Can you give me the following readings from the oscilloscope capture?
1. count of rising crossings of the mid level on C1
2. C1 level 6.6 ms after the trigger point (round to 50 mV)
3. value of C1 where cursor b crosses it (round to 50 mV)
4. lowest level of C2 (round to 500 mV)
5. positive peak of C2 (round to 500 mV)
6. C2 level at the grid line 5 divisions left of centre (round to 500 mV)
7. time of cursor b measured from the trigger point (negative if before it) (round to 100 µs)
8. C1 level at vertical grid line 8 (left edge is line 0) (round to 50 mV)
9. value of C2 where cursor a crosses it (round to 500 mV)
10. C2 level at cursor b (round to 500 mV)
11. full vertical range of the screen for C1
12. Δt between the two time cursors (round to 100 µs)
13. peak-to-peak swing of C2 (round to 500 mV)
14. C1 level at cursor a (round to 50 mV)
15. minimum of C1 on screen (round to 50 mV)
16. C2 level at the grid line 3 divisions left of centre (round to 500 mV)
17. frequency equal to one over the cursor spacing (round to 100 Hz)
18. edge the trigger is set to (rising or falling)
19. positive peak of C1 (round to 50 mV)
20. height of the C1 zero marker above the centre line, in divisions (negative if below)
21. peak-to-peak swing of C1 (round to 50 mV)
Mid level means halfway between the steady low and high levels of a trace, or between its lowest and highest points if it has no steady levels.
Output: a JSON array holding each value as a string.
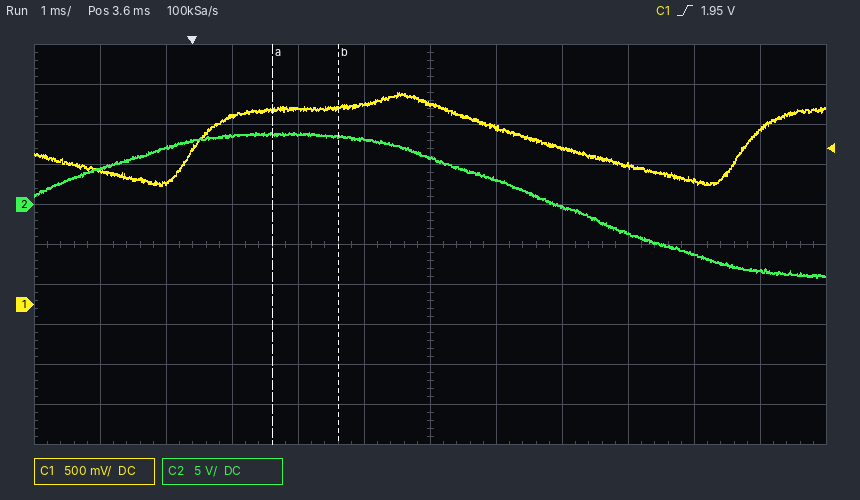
["2", "1.75 V", "2.45 V", "-9.0 V", "9.0 V", "4.5 V", "+2.2 ms", "1.95 V", "9.0 V", "8.5 V", "5 V", "1.0 ms", "18.0 V", "2.45 V", "1.50 V", "8.5 V", "1.0 kHz", "rising", "2.65 V", "-1.5 div", "1.15 V"]
